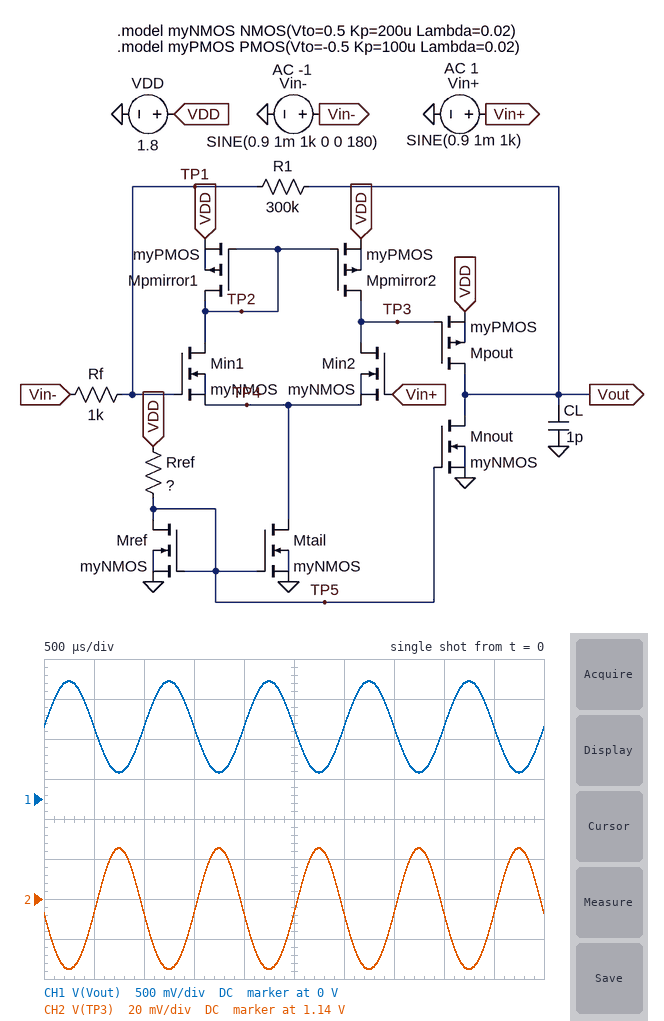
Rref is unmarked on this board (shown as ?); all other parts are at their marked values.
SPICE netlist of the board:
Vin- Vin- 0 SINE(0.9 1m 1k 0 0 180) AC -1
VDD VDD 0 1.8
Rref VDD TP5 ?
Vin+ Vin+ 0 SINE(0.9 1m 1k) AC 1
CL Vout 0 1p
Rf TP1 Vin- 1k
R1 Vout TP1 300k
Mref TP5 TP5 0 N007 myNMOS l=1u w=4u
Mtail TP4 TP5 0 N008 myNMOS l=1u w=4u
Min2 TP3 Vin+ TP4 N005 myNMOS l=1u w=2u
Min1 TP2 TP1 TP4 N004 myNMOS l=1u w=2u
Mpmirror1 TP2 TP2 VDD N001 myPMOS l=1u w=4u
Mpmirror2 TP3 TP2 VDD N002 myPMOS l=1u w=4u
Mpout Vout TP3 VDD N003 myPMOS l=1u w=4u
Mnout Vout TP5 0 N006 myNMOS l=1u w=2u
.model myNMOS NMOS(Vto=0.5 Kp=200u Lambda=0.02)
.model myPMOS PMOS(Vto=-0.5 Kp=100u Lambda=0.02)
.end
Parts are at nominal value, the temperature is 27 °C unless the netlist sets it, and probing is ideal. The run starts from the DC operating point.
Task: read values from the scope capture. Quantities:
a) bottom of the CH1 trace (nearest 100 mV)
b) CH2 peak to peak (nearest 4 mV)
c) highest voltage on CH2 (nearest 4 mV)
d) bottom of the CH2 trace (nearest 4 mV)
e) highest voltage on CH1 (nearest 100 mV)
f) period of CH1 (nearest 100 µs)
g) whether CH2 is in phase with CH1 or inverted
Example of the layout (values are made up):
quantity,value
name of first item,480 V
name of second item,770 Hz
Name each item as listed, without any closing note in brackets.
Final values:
quantity,value
bottom of the CH1 trace,300 mV
CH2 peak to peak,60 mV
highest voltage on CH2,1.164 V
bottom of the CH2 trace,1.104 V
highest voltage on CH1,1.5 V
period of CH1,1.0 ms
whether CH2 is in phase with CH1 or inverted,inverted
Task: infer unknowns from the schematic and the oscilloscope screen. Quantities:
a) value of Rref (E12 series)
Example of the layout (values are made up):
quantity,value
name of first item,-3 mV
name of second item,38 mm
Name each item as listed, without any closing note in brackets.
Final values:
quantity,value
value of Rref,100 kΩ
